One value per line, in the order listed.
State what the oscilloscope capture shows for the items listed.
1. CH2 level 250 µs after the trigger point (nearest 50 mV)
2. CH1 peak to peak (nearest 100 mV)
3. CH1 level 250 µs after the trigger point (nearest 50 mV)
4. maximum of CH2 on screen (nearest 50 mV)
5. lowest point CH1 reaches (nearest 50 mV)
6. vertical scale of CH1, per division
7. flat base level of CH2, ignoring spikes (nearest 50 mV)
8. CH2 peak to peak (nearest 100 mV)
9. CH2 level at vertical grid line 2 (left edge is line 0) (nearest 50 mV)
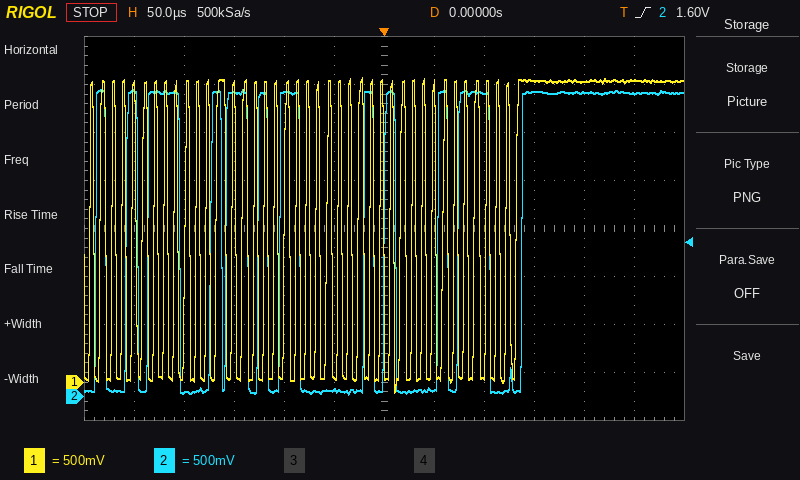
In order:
3.15 V
3.30 V
3.15 V
3.20 V
-100 mV
500 mV
50 mV
3.20 V
50 mV
